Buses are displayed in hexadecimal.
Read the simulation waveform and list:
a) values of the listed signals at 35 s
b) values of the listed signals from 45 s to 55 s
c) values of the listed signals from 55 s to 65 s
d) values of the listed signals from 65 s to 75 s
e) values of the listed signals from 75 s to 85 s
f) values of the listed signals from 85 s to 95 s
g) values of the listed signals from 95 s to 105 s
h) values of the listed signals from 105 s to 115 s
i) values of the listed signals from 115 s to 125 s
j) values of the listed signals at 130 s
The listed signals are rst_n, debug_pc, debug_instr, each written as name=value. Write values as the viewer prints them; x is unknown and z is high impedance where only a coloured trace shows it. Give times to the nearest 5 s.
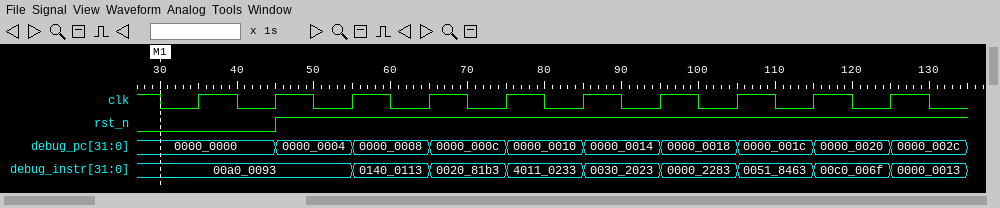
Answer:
rst_n=0, debug_pc=0000_0000, debug_instr=00a0_0093
rst_n=1, debug_pc=0000_0004, debug_instr=00a0_0093
rst_n=1, debug_pc=0000_0008, debug_instr=0140_0113
rst_n=1, debug_pc=0000_000c, debug_instr=0020_81b3
rst_n=1, debug_pc=0000_0010, debug_instr=4011_0233
rst_n=1, debug_pc=0000_0014, debug_instr=0030_2023
rst_n=1, debug_pc=0000_0018, debug_instr=0000_2283
rst_n=1, debug_pc=0000_001c, debug_instr=0051_8463
rst_n=1, debug_pc=0000_0020, debug_instr=00c0_006f
rst_n=1, debug_pc=0000_002c, debug_instr=0000_0013
